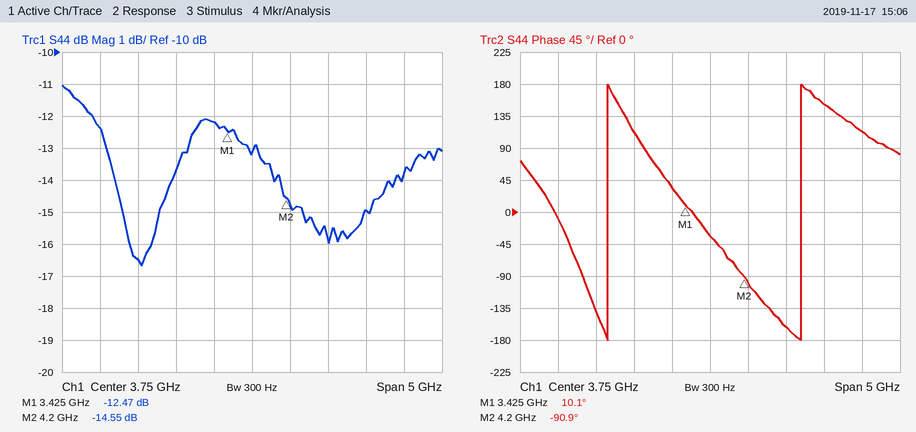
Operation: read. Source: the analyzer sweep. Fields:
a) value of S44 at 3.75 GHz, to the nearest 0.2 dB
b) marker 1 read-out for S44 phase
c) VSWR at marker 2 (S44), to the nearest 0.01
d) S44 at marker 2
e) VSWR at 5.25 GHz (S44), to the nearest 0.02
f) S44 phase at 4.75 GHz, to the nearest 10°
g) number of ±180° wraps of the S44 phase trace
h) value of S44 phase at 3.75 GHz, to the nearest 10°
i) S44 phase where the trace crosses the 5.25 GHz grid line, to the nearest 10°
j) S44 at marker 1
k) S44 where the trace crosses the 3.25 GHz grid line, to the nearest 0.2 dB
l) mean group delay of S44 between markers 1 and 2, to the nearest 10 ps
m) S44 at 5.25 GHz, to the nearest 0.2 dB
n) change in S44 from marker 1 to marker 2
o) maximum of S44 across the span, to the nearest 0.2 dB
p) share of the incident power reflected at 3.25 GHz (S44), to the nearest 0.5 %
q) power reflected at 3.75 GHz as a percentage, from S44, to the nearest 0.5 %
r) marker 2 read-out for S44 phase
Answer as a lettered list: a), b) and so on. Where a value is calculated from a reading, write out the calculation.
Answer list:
a) -13.2 dB
b) 10.1°
c) (1 + 0.1873)/(1 − 0.1873) ≈ 1.46
d) -14.55 dB
e) |Γ| = 10^(-15/20) = 0.1778; VSWR = (1 + 0.1778)/(1 − 0.1778) ≈ 1.43, so 1.44 to the nearest 0.02
f) -160°
g) 2
h) -30°
i) 150°
j) -12.47 dB
k) -12.2 dB
l) −(-90.9° − (10.1°))/(360° × 775 MHz) ≈ 362 ps, so 360 ps to the nearest 10 ps
m) -15.0 dB
n) -14.55 − (-12.47) = -2.08 dB
o) -11.0 dB
p) 10^(-12.2/10) ≈ 6.0 %
q) 10^(-13.2/10) ≈ 4.79 %, so 5.0 % to the nearest 0.5 %
r) -90.9°
